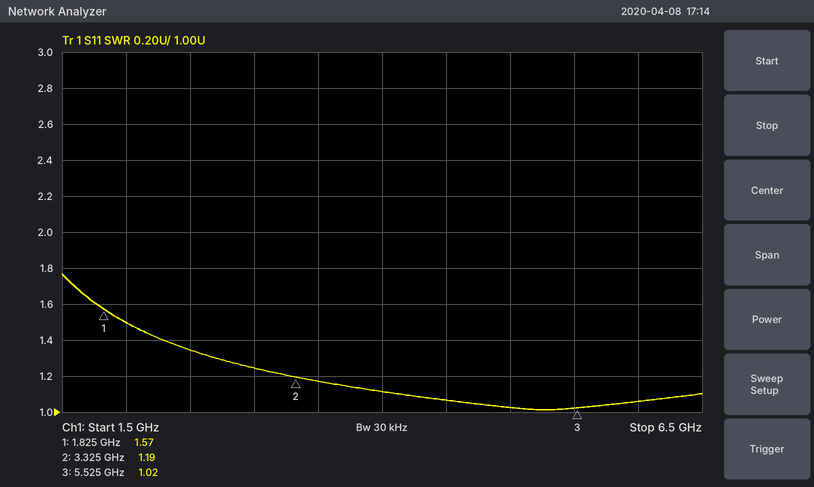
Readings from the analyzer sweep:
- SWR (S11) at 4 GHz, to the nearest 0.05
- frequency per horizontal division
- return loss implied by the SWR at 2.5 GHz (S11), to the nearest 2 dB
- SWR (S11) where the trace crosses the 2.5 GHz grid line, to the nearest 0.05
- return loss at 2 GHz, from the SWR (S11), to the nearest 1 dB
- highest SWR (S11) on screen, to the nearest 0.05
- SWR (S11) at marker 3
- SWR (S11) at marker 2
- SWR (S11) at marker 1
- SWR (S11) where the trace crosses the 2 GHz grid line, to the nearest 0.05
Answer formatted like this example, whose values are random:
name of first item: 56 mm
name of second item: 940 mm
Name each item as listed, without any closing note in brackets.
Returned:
SWR (S11) at 4 GHz, to the nearest 0.05: 1.10
frequency per horizontal division: 500 MHz
return loss implied by the SWR at 2.5 GHz (S11), to the nearest 2 dB: 16 dB
SWR (S11) where the trace crosses the 2.5 GHz grid line, to the nearest 0.05: 1.35
return loss at 2 GHz, from the SWR (S11), to the nearest 1 dB: 14 dB
highest SWR (S11) on screen, to the nearest 0.05: 1.75
SWR (S11) at marker 3: 1.02
SWR (S11) at marker 2: 1.19
SWR (S11) at marker 1: 1.57
SWR (S11) where the trace crosses the 2 GHz grid line, to the nearest 0.05: 1.50
